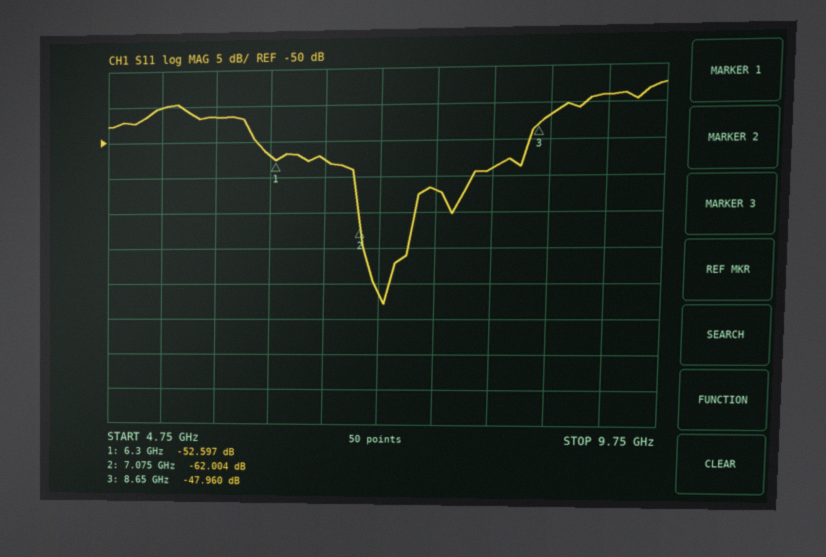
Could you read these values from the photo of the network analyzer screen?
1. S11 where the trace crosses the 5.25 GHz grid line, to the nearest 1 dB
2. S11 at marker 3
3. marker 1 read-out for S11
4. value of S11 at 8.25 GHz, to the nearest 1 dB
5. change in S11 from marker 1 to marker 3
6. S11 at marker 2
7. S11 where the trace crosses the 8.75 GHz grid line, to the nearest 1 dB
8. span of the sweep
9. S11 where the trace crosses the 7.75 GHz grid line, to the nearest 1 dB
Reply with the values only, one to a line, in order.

-45 dB
-47.960 dB
-52.597 dB
-54 dB
4.637 dB
-62.004 dB
-47 dB
5 GHz
-57 dB
